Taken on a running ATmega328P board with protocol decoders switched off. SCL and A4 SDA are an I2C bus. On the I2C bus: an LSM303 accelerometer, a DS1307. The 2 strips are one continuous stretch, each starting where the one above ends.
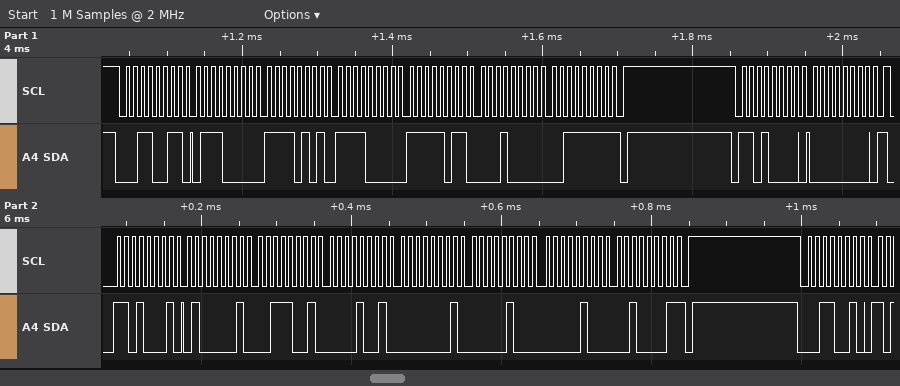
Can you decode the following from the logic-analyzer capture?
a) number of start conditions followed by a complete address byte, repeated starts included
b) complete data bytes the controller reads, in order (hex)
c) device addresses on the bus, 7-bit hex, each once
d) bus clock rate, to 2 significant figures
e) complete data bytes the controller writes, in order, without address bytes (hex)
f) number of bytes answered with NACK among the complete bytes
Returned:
4
70 F5 F0 FB 10 3F 41 39 09 01 04 04 21
0x19 0x68
100 kHz
00
2
